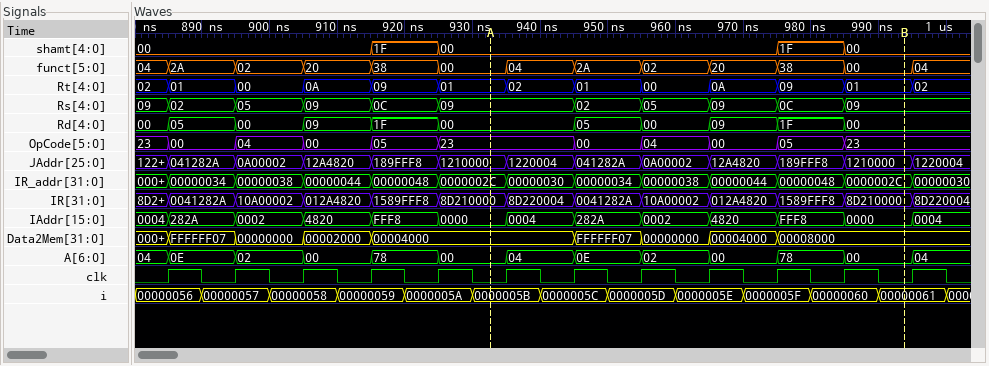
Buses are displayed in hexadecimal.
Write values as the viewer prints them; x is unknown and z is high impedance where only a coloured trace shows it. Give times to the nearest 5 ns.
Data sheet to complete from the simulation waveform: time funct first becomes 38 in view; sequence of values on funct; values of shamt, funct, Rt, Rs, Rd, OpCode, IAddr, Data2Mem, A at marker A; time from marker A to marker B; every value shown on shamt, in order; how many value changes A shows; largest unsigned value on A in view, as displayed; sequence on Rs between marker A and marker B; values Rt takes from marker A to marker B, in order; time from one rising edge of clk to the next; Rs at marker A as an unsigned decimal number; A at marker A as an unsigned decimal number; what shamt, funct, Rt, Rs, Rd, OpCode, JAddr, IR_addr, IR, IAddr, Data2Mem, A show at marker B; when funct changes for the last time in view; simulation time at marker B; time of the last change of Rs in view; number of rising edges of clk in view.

915 ns
04, 2A, 02, 20, 38, 00, 04, 2A, 02, 20, 38, 00, 04
shamt=00, funct=00, Rt=01, Rs=09, Rd=00, OpCode=23, IAddr=0000, Data2Mem=00004000, A=00
60 ns
00, 1F, 00, 1F, 00
12
78
09, 02, 05, 09, 0C, 09
01, 02, 01, 00, 0A, 09, 01
10 ns
9
0
shamt=00, funct=00, Rt=01, Rs=09, Rd=00, OpCode=23, JAddr=1210000, IR_addr=0000002C, IR=8D210000, IAddr=0000, Data2Mem=00008000, A=00
995 ns
995 ns
985 ns
12
